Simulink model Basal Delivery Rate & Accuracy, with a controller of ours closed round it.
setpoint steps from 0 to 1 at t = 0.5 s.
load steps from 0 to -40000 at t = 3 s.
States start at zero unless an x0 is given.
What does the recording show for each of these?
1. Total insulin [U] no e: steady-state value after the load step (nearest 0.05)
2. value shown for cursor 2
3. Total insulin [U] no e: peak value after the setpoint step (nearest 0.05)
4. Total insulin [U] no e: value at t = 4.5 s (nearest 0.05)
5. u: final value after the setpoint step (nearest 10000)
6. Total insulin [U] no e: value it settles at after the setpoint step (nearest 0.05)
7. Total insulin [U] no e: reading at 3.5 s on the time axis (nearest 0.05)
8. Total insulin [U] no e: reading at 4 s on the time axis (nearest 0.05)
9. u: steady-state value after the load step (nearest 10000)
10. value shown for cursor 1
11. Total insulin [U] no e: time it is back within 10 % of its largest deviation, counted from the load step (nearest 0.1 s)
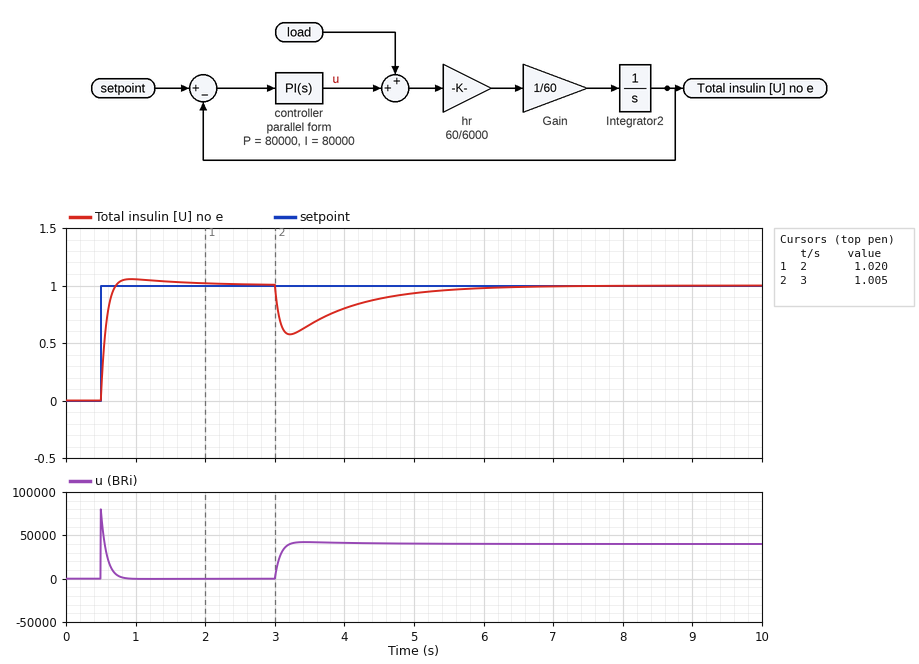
1.00
1.005
1.05
0.90
0
1.00
0.65
0.80
40000
1.020
2.4 s
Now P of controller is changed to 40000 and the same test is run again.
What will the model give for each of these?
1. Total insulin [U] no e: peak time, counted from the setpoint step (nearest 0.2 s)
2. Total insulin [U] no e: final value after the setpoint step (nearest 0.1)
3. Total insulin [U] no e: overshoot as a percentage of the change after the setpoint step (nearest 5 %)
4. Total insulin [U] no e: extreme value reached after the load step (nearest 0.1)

0.6 s
1.0
15 %
0.3
